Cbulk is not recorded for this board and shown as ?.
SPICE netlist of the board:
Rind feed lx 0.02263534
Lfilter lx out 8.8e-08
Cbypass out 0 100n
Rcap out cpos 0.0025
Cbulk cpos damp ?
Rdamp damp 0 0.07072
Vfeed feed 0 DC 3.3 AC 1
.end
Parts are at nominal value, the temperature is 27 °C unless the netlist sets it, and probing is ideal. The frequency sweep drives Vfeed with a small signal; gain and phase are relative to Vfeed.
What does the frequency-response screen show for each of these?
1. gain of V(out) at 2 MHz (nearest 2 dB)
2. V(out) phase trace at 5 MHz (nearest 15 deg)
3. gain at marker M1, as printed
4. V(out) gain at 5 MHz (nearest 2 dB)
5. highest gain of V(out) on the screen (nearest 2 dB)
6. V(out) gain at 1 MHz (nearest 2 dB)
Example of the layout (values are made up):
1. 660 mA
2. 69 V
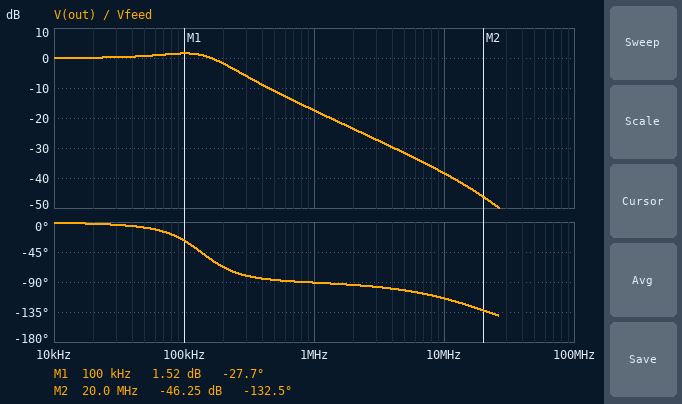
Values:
1. -24 dB
2. -105 deg
3. 1.52 dB
4. -32 dB
5. 2 dB
6. -18 dB
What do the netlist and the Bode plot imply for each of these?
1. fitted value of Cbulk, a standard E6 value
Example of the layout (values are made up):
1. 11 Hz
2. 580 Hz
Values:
1. 15 µF
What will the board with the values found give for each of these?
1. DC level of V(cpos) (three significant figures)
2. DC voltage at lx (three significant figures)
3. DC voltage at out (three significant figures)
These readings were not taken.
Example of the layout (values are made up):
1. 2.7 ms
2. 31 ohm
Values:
1. 3.30 V
2. 3.30 V
3. 3.30 V
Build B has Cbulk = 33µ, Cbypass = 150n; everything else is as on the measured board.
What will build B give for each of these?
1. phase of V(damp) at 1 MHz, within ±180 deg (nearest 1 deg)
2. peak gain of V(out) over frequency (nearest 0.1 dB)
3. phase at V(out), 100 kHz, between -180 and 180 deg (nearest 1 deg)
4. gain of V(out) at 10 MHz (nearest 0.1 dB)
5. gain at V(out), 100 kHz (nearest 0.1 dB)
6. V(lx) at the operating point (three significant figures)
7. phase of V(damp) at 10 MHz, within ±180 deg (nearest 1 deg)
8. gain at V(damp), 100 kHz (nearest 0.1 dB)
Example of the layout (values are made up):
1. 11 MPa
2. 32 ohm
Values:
1. -84 deg
2. 0.2 dB
3. -38 deg
4. -39.2 dB
5. -0.8 dB
6. 3.30 V
7. -124 deg
8. -2.6 dB
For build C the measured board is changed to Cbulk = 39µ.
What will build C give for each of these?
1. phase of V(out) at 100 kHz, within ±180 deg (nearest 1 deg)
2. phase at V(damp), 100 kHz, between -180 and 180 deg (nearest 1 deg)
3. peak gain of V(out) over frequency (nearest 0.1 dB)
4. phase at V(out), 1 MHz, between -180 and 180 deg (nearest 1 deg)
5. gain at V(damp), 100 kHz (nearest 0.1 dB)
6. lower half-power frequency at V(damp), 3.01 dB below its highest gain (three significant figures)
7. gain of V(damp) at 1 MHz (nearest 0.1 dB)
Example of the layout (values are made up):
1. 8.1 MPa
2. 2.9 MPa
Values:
1. -38 deg
2. -9 deg
3. 0.1 dB
4. -86 deg
5. -2.7 dB
6. 35.4 kHz
7. -17.9 dB
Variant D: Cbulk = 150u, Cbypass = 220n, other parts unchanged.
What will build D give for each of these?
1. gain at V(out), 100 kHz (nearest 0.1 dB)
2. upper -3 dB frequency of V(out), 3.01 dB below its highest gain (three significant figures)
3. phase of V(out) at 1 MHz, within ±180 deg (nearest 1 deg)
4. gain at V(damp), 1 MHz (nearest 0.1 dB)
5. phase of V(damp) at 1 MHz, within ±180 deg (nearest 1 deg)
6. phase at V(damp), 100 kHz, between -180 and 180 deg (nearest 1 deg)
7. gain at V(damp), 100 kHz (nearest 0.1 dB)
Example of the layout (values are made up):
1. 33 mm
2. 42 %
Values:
1. -3.1 dB
2. 97.3 kHz
3. -87 deg
4. -17.9 dB
5. -86 deg
6. -25 deg
7. -3.5 dB
